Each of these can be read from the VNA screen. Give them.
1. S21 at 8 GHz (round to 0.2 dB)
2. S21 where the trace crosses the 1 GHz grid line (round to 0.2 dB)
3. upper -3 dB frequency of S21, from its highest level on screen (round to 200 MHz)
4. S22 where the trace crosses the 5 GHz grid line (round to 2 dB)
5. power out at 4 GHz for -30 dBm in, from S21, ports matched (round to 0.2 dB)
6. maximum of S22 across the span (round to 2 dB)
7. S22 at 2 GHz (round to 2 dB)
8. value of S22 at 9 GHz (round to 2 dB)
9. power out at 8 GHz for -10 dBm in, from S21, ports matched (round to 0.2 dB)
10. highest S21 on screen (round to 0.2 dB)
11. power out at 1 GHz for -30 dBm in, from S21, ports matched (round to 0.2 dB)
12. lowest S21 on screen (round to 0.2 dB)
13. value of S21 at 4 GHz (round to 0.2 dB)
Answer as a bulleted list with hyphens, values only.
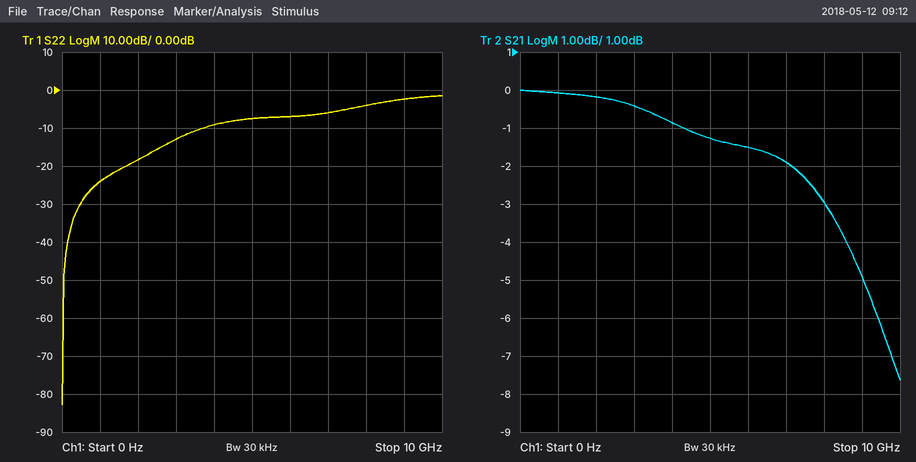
- -3.0 dB
- 0.0 dB
- 8.0 GHz
- -8 dB
- -30.8 dBm
- -2 dB
- -18 dB
- -2 dB
- -13.0 dBm
- 0.0 dB
- -30.0 dBm
- -7.6 dB
- -0.8 dB
